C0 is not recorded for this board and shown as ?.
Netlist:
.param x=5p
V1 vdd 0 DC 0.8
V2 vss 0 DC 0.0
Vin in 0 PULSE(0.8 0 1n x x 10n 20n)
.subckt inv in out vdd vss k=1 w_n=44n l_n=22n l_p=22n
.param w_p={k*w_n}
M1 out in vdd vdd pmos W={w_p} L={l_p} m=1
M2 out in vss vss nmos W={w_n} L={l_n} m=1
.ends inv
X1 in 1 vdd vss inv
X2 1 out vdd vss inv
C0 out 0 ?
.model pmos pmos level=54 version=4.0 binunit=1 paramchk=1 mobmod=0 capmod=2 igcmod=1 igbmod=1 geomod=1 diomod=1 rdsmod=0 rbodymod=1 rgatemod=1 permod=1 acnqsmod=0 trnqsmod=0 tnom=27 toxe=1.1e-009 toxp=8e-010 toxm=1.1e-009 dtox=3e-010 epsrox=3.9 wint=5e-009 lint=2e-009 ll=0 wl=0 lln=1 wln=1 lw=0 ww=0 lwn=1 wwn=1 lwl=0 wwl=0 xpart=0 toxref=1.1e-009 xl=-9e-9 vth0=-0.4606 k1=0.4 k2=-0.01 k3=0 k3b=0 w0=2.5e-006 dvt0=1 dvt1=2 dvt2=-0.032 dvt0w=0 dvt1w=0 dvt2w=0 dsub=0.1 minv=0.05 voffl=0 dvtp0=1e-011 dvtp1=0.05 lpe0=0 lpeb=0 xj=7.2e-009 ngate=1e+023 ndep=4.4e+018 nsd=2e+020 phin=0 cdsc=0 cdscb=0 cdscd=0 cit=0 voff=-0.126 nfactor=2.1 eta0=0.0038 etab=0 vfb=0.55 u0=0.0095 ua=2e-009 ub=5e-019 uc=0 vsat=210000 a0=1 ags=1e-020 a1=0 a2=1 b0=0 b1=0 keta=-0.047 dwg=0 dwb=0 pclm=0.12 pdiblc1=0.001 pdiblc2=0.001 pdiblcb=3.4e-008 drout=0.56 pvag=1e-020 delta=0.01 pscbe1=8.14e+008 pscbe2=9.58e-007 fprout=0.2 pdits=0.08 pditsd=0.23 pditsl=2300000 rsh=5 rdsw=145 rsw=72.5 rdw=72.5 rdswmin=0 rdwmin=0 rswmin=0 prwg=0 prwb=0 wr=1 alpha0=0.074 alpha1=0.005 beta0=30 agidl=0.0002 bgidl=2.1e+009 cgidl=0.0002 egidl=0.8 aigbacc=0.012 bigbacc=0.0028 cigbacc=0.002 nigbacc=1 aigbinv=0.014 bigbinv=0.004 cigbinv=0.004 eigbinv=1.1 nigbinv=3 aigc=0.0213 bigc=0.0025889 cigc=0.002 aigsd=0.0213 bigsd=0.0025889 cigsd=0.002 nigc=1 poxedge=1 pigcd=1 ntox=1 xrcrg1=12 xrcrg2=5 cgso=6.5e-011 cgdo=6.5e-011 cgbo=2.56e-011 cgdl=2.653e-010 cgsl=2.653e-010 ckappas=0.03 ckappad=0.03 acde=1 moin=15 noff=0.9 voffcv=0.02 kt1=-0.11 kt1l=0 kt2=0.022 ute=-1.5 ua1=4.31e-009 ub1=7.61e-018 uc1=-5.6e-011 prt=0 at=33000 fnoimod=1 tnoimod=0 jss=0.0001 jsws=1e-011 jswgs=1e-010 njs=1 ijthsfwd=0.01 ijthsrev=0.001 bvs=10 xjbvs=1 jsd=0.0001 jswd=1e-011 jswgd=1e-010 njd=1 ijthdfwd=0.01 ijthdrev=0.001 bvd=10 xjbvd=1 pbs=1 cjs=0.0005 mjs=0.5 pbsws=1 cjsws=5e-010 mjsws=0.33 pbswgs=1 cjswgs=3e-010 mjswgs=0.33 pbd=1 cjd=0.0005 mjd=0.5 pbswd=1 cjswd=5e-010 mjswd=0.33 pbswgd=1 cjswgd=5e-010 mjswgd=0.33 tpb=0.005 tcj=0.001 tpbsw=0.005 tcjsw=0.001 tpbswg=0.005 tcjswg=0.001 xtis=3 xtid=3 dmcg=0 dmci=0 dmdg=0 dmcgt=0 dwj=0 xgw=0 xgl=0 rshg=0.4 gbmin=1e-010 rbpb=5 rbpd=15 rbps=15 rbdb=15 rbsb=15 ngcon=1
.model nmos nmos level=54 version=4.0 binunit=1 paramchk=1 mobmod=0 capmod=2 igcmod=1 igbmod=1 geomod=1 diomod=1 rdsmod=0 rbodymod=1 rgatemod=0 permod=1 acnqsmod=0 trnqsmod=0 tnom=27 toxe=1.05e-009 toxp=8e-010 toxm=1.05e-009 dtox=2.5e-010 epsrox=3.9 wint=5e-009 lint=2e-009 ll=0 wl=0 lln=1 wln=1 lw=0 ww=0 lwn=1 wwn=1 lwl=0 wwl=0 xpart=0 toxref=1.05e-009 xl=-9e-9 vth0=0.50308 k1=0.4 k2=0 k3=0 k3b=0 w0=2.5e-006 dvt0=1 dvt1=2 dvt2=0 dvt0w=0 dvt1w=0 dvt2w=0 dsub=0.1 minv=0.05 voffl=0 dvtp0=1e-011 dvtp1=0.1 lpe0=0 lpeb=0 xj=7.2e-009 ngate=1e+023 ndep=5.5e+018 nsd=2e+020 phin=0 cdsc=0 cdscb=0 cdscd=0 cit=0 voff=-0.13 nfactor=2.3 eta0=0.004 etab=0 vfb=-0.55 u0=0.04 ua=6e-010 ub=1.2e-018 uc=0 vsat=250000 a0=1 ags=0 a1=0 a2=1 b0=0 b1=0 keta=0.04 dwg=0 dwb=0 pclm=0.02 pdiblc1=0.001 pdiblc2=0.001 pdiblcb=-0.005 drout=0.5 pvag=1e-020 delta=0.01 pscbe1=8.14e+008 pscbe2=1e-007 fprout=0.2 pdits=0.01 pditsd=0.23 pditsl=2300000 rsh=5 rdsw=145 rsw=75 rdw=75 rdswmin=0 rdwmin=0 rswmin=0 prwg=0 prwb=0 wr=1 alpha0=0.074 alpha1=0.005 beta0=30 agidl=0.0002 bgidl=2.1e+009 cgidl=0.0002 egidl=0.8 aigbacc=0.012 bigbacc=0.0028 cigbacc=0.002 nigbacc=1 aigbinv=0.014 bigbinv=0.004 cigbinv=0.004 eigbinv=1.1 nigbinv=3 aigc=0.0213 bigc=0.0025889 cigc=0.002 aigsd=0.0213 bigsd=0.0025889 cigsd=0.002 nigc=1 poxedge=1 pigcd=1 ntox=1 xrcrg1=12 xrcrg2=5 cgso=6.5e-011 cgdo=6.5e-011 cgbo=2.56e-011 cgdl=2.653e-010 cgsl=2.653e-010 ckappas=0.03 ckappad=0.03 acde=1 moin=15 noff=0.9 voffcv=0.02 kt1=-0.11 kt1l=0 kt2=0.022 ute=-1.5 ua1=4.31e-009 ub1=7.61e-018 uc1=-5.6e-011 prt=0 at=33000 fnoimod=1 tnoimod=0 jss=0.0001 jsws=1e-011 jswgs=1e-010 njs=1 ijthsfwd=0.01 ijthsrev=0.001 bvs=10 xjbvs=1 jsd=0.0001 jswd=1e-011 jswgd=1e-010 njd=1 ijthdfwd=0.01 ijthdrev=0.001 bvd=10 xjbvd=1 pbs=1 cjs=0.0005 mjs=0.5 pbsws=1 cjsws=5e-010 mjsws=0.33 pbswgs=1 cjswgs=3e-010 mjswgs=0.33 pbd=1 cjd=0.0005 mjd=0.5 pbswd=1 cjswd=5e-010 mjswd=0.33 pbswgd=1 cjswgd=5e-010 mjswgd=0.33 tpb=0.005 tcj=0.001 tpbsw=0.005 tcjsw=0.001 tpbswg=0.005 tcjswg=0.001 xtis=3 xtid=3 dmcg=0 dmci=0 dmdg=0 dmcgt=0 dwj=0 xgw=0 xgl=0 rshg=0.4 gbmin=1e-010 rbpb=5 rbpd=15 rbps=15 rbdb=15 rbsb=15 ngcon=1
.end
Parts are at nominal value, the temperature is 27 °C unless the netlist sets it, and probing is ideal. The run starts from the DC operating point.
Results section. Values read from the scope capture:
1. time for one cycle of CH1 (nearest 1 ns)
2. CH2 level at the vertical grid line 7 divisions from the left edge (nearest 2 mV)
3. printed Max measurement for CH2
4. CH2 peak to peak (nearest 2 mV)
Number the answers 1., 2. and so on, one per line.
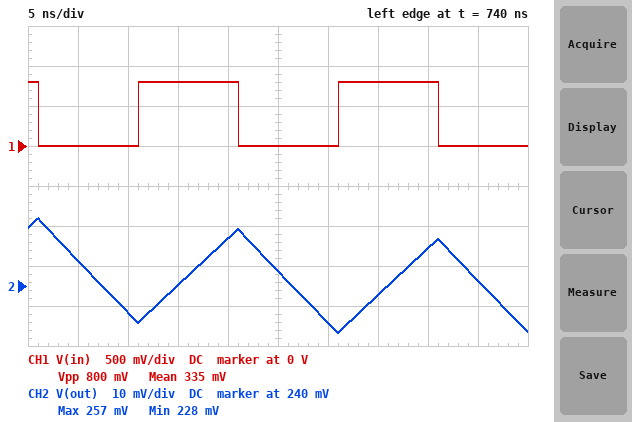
1. 20 ns
2. 238 mV
3. 257 mV
4. 28 mV
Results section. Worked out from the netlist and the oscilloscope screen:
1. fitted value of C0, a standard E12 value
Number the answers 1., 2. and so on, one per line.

1. 12 pF
